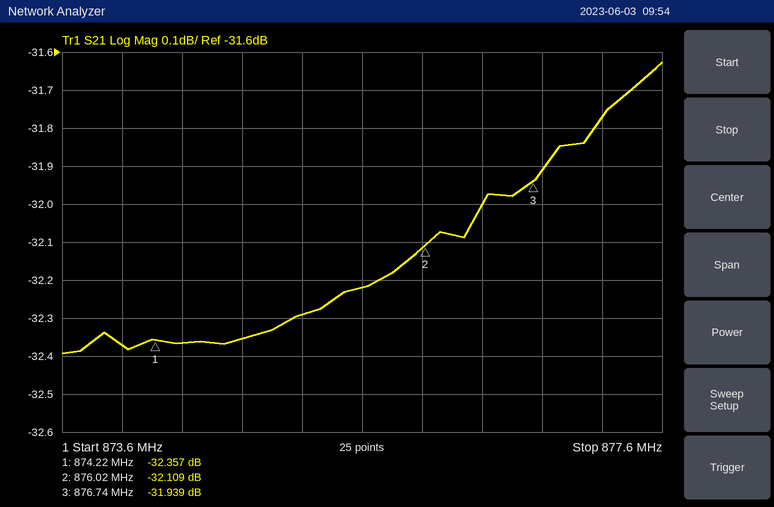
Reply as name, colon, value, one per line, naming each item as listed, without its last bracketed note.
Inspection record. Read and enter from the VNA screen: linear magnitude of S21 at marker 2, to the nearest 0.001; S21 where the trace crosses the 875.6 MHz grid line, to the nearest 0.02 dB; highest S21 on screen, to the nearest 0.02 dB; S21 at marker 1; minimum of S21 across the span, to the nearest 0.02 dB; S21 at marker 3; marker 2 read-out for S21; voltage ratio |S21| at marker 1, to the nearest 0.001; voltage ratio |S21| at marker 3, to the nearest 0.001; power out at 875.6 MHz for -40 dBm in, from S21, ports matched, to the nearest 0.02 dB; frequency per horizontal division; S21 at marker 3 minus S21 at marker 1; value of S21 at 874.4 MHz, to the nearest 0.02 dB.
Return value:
linear magnitude of S21 at marker 2, to the nearest 0.001: 0.025
S21 where the trace crosses the 875.6 MHz grid line, to the nearest 0.02 dB: -32.22 dB
highest S21 on screen, to the nearest 0.02 dB: -31.62 dB
S21 at marker 1: -32.357 dB
minimum of S21 across the span, to the nearest 0.02 dB: -32.40 dB
S21 at marker 3: -31.939 dB
marker 2 read-out for S21: -32.109 dB
voltage ratio |S21| at marker 1, to the nearest 0.001: 0.024
voltage ratio |S21| at marker 3, to the nearest 0.001: 0.025
power out at 875.6 MHz for -40 dBm in, from S21, ports matched, to the nearest 0.02 dB: -72.22 dBm
frequency per horizontal division: 400 kHz
S21 at marker 3 minus S21 at marker 1: 0.418 dB
value of S21 at 874.4 MHz, to the nearest 0.02 dB: -32.36 dB
